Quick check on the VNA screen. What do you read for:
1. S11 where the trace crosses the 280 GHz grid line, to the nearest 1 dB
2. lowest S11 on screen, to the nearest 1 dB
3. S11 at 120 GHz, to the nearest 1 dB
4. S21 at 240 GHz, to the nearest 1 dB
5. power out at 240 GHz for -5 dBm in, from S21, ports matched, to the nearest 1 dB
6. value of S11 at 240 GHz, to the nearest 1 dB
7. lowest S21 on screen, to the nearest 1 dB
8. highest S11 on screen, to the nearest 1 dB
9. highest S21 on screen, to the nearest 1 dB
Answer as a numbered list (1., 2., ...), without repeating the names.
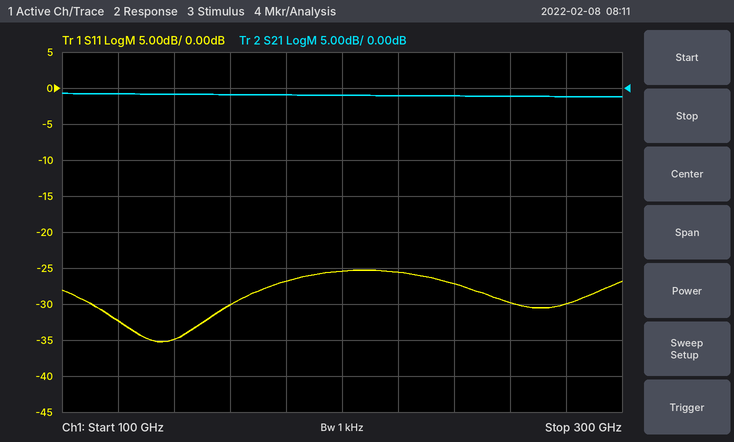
1. -30 dB
2. -35 dB
3. -32 dB
4. -1 dB
5. -6 dBm
6. -27 dB
7. -1 dB
8. -25 dB
9. -1 dB
